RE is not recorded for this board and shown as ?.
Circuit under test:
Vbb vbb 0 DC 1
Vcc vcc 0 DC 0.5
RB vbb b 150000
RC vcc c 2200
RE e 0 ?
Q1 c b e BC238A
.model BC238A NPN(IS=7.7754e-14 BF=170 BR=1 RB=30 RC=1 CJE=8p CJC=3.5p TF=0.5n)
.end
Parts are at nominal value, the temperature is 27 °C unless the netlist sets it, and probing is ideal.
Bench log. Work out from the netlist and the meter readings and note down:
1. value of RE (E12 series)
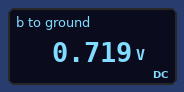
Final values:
1.8 kΩ
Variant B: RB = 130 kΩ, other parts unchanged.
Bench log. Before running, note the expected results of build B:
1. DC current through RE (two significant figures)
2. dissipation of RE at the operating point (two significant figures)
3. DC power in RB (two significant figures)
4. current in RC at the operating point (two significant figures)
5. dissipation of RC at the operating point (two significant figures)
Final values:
99 µA
18 µW
600 nW
97 µA
21 µW
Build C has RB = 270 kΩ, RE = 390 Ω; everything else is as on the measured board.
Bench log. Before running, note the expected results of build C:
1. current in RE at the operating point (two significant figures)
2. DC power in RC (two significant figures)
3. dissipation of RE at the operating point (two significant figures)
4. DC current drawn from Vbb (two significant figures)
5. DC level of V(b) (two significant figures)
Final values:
140 µA
42 µW
7.7 µW
1.5 µA
610 mV
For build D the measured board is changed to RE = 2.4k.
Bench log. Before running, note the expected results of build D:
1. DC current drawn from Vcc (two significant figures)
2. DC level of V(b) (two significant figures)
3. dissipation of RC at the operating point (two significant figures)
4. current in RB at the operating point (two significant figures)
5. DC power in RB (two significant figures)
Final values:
84 µA
740 mV
15 µW
1.7 µA
440 nW
